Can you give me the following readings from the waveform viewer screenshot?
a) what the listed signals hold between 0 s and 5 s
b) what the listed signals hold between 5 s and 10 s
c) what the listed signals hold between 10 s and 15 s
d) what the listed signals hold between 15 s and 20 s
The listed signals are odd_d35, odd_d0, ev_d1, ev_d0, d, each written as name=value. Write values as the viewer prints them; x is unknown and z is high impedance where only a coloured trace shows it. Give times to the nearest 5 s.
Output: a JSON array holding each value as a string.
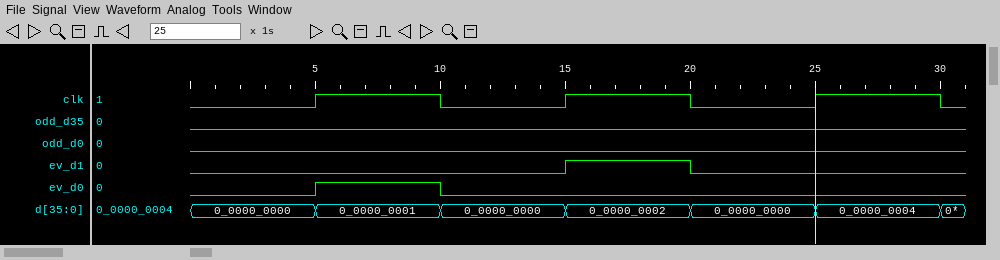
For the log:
["odd_d35=0, odd_d0=0, ev_d1=0, ev_d0=0, d=0_0000_0000", "odd_d35=0, odd_d0=0, ev_d1=0, ev_d0=1, d=0_0000_0001", "odd_d35=0, odd_d0=0, ev_d1=0, ev_d0=0, d=0_0000_0000", "odd_d35=0, odd_d0=0, ev_d1=1, ev_d0=0, d=0_0000_0002"]
